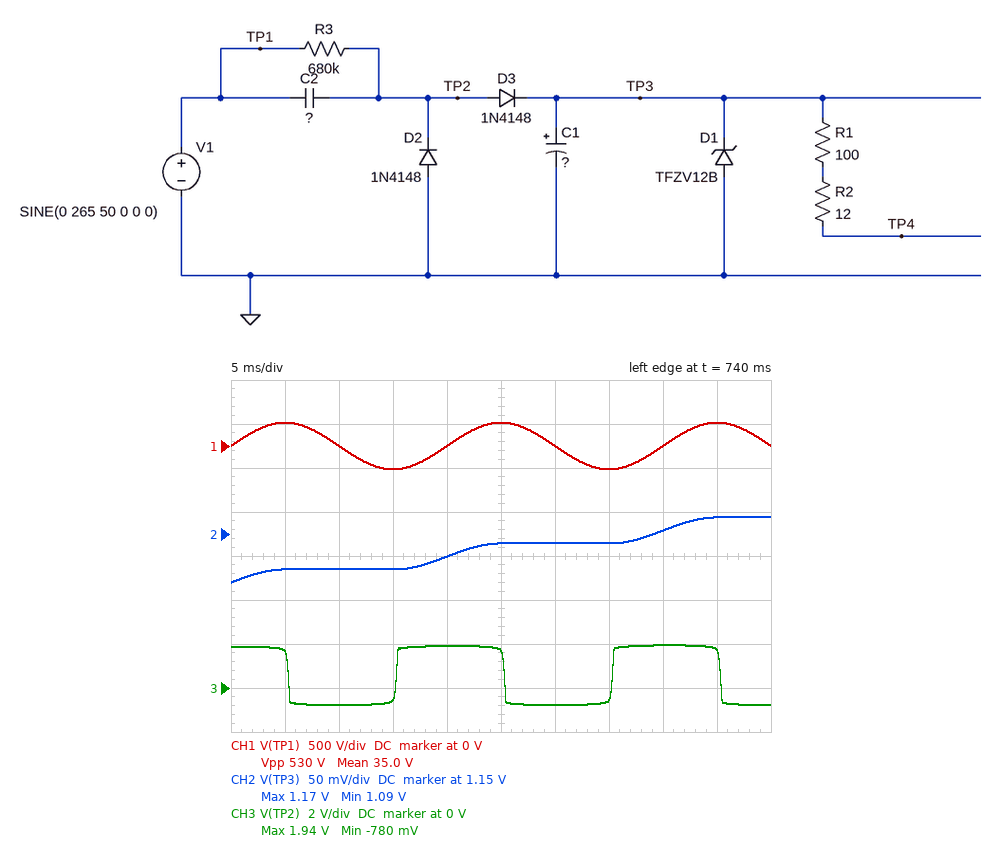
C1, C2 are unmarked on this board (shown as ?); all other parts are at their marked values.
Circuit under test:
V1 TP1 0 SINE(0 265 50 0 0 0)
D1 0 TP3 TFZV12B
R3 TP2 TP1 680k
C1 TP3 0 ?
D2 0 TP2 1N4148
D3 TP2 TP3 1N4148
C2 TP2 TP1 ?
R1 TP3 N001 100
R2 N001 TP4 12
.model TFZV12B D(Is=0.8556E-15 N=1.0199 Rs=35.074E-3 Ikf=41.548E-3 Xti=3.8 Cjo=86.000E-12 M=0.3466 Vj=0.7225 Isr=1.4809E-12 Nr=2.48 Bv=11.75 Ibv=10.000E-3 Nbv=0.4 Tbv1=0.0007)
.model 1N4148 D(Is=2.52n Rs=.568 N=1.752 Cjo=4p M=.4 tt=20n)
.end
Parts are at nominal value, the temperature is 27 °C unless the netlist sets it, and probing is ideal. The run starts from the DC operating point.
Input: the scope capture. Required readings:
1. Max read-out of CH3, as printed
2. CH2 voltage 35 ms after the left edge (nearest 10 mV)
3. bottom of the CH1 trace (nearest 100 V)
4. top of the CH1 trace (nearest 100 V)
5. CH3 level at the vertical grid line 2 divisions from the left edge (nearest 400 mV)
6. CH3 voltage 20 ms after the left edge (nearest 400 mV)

1.94 V
1.14 V
-300 V
300 V
-800 mV
2.0 V
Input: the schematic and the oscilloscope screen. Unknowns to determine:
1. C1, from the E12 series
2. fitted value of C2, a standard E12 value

10 mF
560 nF
